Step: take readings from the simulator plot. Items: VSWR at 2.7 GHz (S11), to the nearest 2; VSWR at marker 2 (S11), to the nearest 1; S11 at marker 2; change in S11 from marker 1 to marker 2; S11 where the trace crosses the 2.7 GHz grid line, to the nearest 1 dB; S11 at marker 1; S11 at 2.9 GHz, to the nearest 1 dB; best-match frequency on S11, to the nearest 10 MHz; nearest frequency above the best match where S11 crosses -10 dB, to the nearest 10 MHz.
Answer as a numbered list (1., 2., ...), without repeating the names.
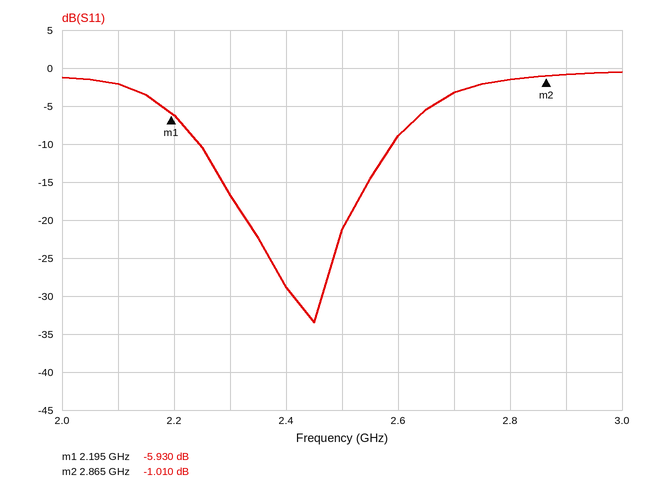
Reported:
1. 6
2. 17
3. -1.010 dB
4. 4.920 dB
5. -3 dB
6. -5.930 dB
7. -1 dB
8. 2.45 GHz
9. 2.59 GHz
